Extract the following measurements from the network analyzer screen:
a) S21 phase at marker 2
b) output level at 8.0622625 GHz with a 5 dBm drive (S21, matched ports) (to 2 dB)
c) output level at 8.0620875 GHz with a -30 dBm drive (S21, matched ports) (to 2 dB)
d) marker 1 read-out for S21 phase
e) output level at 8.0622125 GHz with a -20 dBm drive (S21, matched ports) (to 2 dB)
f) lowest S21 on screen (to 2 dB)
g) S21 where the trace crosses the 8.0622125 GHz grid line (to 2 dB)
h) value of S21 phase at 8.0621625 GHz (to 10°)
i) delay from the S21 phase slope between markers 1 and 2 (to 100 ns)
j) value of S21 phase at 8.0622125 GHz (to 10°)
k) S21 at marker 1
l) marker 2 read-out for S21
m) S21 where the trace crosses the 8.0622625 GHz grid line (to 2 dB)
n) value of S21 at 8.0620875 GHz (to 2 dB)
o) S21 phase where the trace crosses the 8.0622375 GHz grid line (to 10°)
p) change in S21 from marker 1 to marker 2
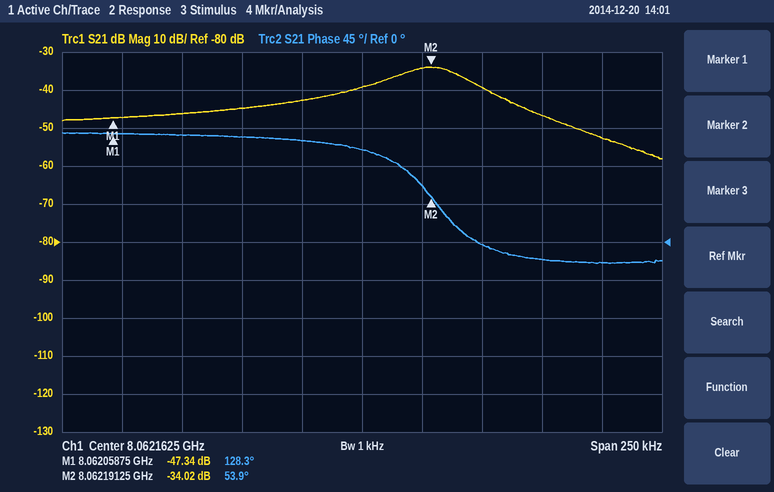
53.9°
-48 dBm
-76 dBm
128.3°
-60 dBm
-58 dB
-40 dB
110°
1.6 µs
0°
-47.34 dB
-34.02 dB
-52 dB
-46 dB
-20°
13.32 dB
